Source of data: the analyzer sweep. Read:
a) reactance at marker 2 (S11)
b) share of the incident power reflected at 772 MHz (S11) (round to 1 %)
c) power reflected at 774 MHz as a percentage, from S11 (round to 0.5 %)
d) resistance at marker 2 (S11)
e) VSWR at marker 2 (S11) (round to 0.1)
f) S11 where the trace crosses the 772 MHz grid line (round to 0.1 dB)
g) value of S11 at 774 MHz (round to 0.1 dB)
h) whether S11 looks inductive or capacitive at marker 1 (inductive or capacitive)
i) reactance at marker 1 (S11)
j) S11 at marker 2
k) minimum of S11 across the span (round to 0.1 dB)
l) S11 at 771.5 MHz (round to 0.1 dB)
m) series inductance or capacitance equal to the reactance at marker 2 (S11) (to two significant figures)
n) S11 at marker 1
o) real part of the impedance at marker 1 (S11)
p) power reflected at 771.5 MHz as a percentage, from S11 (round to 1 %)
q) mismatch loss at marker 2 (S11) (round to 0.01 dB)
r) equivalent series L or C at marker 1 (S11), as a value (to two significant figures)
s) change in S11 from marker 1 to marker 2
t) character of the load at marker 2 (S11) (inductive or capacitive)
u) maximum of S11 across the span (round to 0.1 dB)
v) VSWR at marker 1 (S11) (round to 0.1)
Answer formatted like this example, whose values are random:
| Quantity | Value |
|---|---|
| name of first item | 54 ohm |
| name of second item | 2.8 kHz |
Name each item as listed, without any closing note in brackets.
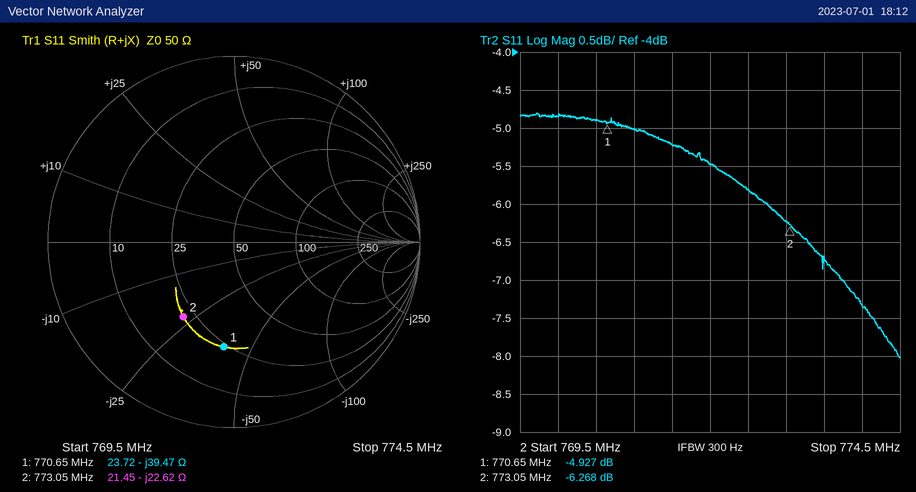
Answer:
| Quantity | Value |
|---|---|
| reactance at marker 2 | -22.62 Ω |
| share of the incident power reflected at 772 MHz (S11) | 28 % |
| power reflected at 774 MHz as a percentage, from S11 | 18.5 % |
| resistance at marker 2 | 21.45 Ω |
| VSWR at marker 2 (S11) | 2.9 |
| S11 where the trace crosses the 772 MHz grid line | -5.5 dB |
| value of S11 at 774 MHz | -7.3 dB |
| whether S11 looks inductive or capacitive at marker 1 | capacitive |
| reactance at marker 1 | -39.47 Ω |
| S11 at marker 2 | -6.268 dB |
| minimum of S11 across the span | -8.0 dB |
| S11 at 771.5 MHz | -5.2 dB |
| series inductance or capacitance equal to the reactance at marker 2 (S11) | 9.1 pF |
| S11 at marker 1 | -4.927 dB |
| real part of the impedance at marker 1 | 23.72 Ω |
| power reflected at 771.5 MHz as a percentage, from S11 | 30 % |
| mismatch loss at marker 2 (S11) | 1.17 dB |
| equivalent series L or C at marker 1 (S11), as a value | 5.2 pF |
| change in S11 from marker 1 to marker 2 | -1.341 dB |
| character of the load at marker 2 (S11) | capacitive |
| maximum of S11 across the span | -4.8 dB |
| VSWR at marker 1 (S11) | 3.6 |
